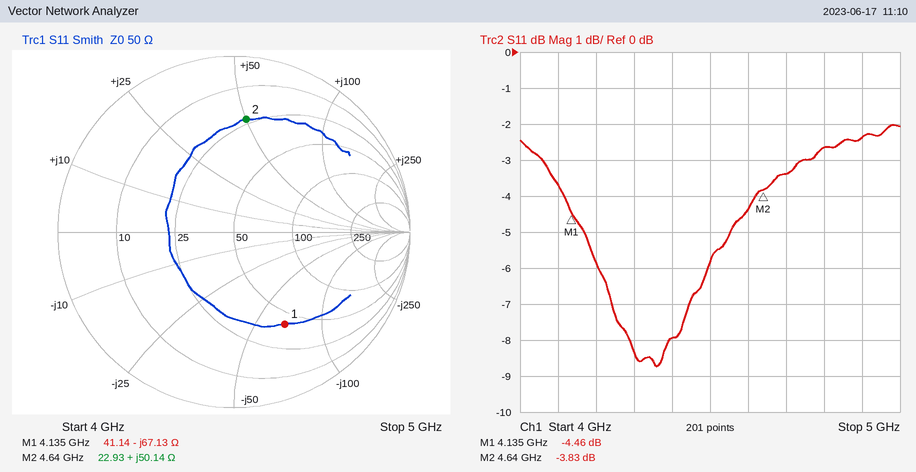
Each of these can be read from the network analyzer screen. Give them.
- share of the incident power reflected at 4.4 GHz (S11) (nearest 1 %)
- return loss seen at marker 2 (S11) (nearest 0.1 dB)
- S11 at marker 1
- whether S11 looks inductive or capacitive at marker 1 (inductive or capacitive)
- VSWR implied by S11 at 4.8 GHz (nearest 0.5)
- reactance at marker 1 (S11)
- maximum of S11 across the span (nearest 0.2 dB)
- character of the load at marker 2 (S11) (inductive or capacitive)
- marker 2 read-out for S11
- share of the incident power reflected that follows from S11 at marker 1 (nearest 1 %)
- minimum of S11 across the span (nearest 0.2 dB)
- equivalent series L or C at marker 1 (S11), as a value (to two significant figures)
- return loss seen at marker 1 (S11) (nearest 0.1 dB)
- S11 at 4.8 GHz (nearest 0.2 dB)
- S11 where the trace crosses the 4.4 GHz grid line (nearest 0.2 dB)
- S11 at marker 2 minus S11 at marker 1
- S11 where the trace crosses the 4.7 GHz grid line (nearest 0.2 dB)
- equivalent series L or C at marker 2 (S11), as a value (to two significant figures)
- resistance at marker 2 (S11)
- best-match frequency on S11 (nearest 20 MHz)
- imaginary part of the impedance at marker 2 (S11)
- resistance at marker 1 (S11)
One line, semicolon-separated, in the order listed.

16 %; 3.8 dB; -4.46 dB; capacitive; 6.5; -67.13 Ω; -2.0 dB; inductive; -3.83 dB; 36 %; -8.8 dB; 570 fF; 4.5 dB; -2.6 dB; -8.0 dB; 0.63 dB; -3.4 dB; 1.7 nH; 22.93 Ω; 4.36 GHz; +50.14 Ω; 41.14 Ω
